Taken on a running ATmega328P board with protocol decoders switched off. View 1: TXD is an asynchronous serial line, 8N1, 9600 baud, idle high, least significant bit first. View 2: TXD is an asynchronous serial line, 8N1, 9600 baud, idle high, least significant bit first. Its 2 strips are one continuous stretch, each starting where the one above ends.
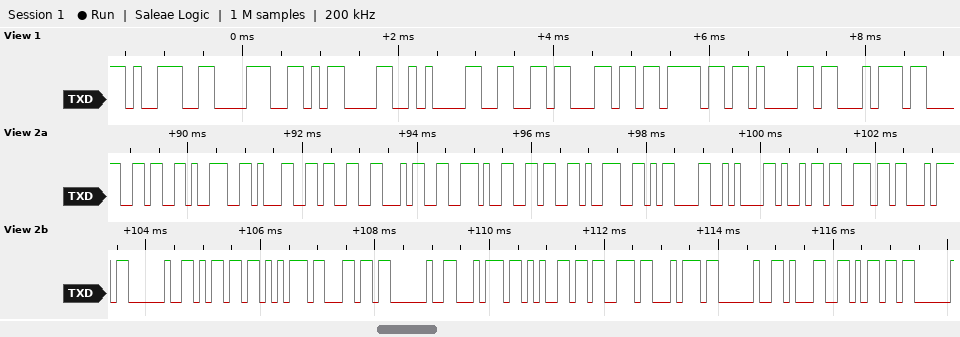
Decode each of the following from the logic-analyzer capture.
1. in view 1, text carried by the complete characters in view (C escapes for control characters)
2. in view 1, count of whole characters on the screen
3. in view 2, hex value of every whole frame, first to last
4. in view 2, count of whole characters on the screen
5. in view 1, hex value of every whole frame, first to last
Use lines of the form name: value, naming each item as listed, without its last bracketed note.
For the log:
in view 1, text carried by the complete characters in view: "98\r\nfloat"
in view 1, count of whole characters on the screen: 9
in view 2, hex value of every whole frame, first to last: 36 39 31 33 34 2E 36 39 0D 0A 69 6E 74 20 6D 75 6C 20 74 65 73 74 20 31 6D
in view 2, count of whole characters on the screen: 25
in view 1, hex value of every whole frame, first to last: 39 38 0D 0A 66 6C 6F 61 74
